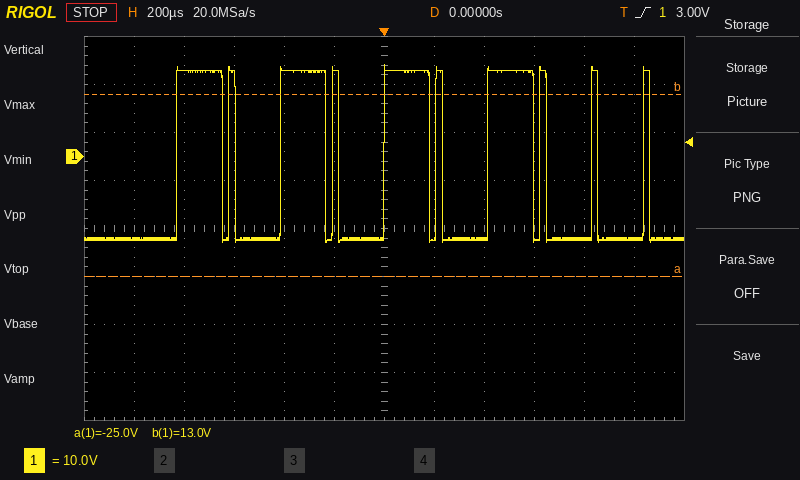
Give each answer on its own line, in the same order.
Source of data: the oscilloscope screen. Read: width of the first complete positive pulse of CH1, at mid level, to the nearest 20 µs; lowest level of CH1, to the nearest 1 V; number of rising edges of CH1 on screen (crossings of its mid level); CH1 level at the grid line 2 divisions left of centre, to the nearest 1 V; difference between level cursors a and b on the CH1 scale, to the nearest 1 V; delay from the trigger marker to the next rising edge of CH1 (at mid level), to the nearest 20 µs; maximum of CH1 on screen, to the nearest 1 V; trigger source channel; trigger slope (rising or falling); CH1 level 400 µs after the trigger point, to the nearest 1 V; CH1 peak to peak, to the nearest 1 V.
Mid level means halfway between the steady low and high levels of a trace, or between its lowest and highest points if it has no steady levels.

180 µs
-18 V
10
18 V
38 V
200 µs
19 V
CH1
rising
-17 V
37 V
